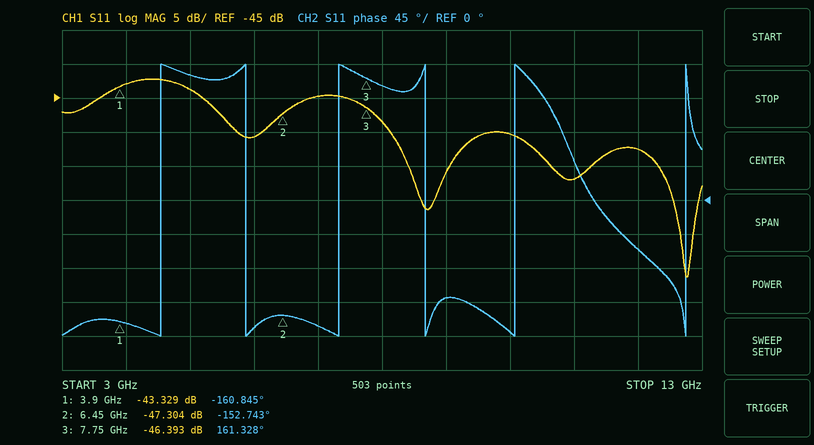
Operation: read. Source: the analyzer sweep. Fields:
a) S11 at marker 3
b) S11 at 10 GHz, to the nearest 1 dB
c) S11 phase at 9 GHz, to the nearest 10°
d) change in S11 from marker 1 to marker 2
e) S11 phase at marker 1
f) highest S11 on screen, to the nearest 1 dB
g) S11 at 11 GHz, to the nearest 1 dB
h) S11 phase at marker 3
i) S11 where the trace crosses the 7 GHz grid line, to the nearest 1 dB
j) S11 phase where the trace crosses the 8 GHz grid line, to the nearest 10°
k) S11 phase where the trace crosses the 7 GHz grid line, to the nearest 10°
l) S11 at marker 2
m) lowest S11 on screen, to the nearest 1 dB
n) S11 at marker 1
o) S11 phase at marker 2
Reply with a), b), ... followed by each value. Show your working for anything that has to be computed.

a) -46.393 dB
b) -50 dB
c) -130°
d) -47.304 − (-43.329) = -3.975 dB
e) -160.845°
f) -42 dB
g) -57 dB
h) 161.328°
i) -45 dB
j) 150°
k) -170°
l) -47.304 dB
m) -71 dB
n) -43.329 dB
o) -152.743°
